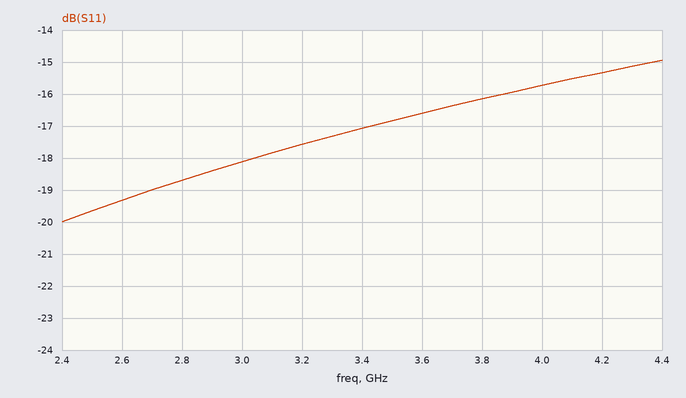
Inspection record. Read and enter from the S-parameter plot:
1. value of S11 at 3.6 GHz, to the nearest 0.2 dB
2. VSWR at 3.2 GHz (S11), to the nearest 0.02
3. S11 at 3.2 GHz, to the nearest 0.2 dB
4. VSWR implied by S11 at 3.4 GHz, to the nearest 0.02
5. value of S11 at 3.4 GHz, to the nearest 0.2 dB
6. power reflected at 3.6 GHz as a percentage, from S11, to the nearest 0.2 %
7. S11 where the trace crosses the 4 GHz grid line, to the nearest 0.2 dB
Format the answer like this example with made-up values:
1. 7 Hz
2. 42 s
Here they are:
1. -16.6 dB
2. 1.30
3. -17.6 dB
4. 1.32
5. -17.0 dB
6. 2.2 %
7. -15.8 dB
